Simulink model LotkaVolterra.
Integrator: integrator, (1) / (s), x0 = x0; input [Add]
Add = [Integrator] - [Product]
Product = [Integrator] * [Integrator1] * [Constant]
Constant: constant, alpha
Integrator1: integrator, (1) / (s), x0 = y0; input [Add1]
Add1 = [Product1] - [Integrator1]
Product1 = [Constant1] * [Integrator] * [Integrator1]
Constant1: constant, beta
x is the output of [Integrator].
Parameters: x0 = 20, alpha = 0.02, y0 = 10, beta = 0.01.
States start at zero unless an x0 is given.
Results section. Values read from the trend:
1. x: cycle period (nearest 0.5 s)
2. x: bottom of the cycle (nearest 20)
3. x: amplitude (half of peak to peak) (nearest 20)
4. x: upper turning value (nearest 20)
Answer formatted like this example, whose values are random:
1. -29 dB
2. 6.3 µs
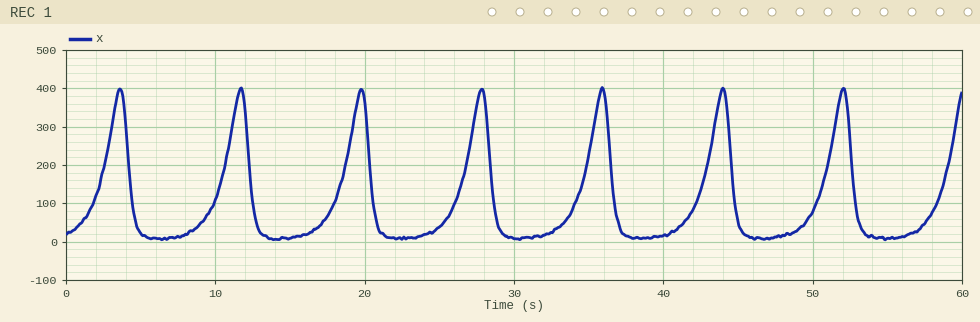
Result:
1. 8.0 s
2. 0
3. 200
4. 400
